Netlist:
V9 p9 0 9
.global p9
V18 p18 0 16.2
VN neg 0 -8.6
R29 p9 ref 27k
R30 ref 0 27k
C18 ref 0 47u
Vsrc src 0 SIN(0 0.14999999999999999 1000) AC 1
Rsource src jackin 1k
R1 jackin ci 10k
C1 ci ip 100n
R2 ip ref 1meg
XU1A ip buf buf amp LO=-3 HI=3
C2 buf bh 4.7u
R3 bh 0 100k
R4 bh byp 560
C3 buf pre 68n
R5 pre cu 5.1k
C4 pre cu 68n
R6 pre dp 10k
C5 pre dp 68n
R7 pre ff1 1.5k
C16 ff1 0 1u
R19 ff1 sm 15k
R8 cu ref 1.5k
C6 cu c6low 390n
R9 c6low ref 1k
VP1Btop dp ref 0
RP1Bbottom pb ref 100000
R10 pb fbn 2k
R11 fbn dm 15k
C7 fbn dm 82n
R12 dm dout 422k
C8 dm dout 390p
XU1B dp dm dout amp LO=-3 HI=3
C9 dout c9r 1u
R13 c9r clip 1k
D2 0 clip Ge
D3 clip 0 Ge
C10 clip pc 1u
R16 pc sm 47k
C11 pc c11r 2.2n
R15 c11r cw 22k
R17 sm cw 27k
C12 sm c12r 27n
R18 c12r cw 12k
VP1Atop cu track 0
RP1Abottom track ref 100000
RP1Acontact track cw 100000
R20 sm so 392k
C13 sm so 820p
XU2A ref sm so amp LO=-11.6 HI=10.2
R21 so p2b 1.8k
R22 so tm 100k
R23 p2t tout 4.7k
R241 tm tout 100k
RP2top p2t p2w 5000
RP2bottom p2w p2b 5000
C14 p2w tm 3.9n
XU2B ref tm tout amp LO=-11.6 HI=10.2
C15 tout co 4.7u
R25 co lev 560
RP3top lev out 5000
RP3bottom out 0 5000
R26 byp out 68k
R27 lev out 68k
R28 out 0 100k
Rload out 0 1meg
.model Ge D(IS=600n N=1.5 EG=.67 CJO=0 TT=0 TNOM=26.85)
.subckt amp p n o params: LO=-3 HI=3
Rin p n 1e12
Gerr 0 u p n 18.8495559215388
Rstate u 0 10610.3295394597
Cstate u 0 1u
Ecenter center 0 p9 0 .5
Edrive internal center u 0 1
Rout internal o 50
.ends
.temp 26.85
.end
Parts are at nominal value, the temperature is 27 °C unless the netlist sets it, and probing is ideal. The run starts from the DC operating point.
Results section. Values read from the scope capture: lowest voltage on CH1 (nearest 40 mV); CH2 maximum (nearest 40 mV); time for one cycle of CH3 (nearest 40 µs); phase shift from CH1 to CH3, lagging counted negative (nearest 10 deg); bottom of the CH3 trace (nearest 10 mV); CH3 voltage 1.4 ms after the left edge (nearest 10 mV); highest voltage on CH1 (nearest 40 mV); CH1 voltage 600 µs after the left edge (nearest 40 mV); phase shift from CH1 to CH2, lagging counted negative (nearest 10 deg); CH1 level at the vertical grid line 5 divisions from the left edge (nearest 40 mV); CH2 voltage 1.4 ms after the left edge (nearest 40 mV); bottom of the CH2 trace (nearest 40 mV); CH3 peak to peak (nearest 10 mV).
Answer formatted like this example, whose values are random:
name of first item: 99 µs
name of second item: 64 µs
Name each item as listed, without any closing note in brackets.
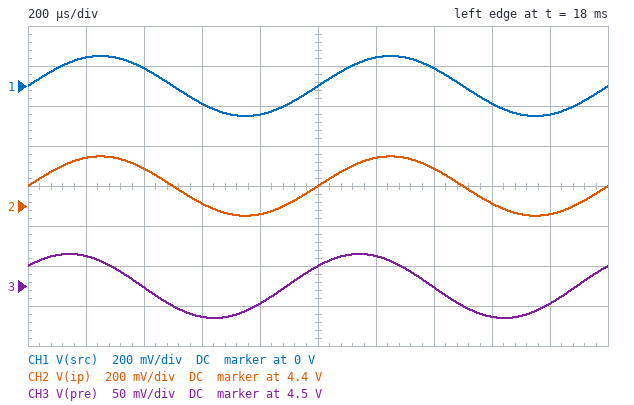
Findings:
lowest voltage on CH1: -160 mV
CH2 maximum: 4.64 V
time for one cycle of CH3: 1.00 ms
phase shift from CH1 to CH3, lagging counted negative: 40 deg
bottom of the CH3 trace: 4.46 V
CH3 voltage 1.4 ms after the left edge: 4.50 V
highest voltage on CH1: 160 mV
CH1 voltage 600 µs after the left edge: -80 mV
phase shift from CH1 to CH2, lagging counted negative: 0 deg
CH1 level at the vertical grid line 5 divisions from the left edge: 0 V
CH2 voltage 1.4 ms after the left edge: 4.60 V
bottom of the CH2 trace: 4.36 V
CH3 peak to peak: 80 mV
